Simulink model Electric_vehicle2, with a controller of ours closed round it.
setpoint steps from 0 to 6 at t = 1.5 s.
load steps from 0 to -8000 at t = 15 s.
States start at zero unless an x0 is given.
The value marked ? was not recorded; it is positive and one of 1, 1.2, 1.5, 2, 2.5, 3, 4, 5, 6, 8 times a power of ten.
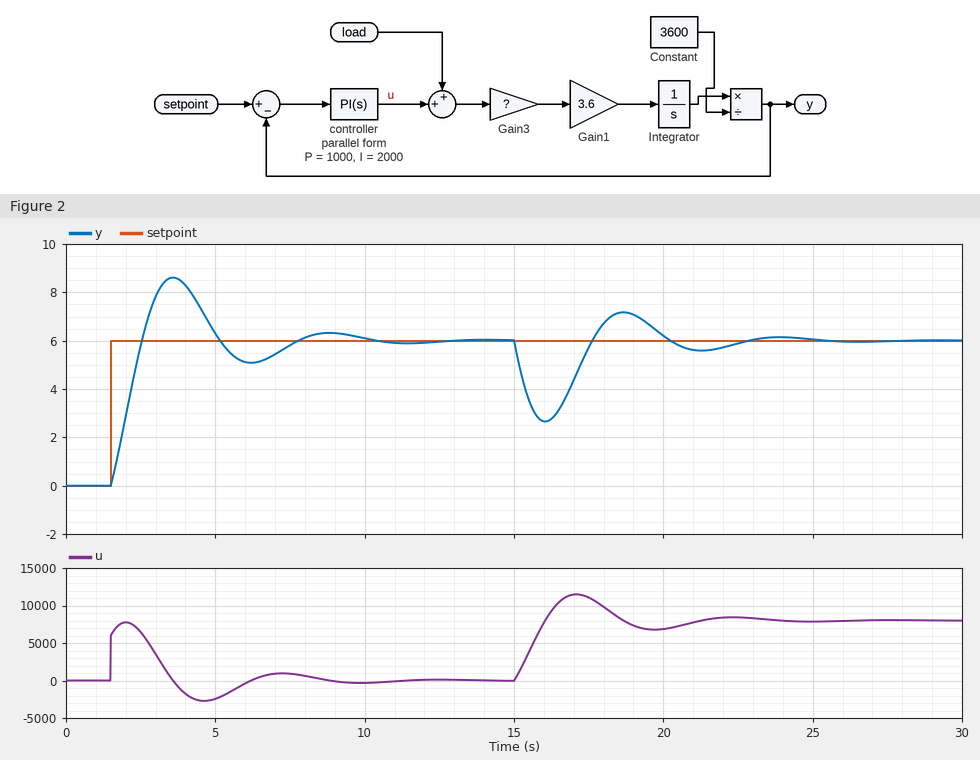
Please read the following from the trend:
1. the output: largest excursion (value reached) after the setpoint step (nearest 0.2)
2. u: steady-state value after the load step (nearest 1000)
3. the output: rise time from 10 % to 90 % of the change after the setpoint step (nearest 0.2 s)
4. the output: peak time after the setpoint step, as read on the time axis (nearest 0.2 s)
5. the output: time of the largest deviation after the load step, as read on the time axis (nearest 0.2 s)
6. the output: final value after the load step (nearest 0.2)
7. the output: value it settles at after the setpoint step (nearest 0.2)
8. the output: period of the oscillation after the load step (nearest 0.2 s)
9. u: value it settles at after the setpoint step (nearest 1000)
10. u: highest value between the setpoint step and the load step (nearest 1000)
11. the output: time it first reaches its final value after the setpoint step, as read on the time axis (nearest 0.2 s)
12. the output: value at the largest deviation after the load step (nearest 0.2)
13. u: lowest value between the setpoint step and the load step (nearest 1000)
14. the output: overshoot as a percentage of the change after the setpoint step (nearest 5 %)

8.6
8000
0.8 s
3.6 s
16.0 s
6.0
6.0
5.2 s
0
8000
2.6 s
2.6
-3000
45 %
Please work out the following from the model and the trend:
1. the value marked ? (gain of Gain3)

0.8
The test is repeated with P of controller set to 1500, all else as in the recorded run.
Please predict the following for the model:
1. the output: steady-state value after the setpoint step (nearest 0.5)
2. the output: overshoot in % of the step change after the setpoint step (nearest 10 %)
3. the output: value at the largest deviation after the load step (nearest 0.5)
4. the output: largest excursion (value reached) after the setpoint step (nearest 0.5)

6.0
30 %
3.0
8.0
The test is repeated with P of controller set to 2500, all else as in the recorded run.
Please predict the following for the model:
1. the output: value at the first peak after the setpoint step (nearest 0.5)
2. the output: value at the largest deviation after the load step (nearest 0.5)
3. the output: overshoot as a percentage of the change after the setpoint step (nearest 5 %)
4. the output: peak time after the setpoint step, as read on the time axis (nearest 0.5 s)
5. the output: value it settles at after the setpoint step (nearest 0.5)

7.0
4.0
20 %
3.0 s
6.0
